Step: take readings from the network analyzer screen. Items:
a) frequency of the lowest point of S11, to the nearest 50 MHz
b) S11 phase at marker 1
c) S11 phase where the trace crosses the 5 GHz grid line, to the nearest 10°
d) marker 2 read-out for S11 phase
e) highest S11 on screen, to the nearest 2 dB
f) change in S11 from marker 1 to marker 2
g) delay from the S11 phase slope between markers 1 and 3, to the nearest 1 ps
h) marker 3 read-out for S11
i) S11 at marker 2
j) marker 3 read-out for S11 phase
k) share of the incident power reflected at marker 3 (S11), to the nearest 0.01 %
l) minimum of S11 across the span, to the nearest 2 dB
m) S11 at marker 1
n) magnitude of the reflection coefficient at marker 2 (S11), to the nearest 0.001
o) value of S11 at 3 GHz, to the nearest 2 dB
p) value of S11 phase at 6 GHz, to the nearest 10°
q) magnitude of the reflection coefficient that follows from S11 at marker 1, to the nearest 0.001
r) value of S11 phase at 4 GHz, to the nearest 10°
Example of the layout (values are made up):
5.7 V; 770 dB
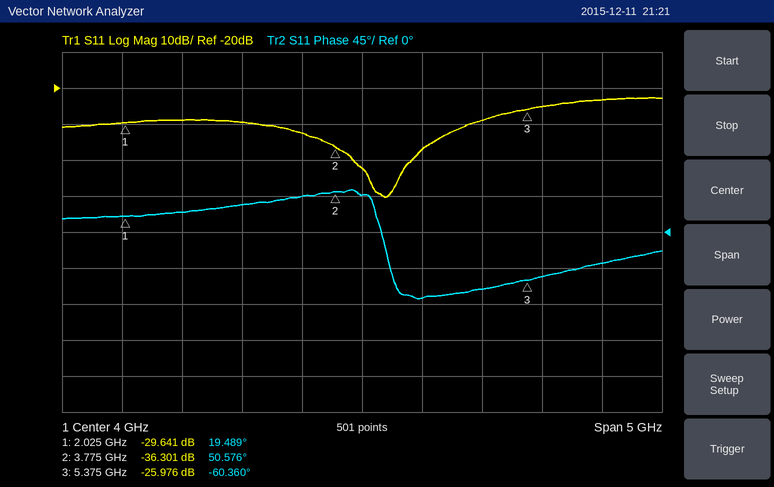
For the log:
4.20 GHz; 19.489°; -70°; 50.576°; -22 dB; -6.660 dB; 66 ps; -25.976 dB; -36.301 dB; -60.360°; 0.25 %; -50 dB; -29.641 dB; 0.015; -30 dB; -40°; 0.033; 50°
